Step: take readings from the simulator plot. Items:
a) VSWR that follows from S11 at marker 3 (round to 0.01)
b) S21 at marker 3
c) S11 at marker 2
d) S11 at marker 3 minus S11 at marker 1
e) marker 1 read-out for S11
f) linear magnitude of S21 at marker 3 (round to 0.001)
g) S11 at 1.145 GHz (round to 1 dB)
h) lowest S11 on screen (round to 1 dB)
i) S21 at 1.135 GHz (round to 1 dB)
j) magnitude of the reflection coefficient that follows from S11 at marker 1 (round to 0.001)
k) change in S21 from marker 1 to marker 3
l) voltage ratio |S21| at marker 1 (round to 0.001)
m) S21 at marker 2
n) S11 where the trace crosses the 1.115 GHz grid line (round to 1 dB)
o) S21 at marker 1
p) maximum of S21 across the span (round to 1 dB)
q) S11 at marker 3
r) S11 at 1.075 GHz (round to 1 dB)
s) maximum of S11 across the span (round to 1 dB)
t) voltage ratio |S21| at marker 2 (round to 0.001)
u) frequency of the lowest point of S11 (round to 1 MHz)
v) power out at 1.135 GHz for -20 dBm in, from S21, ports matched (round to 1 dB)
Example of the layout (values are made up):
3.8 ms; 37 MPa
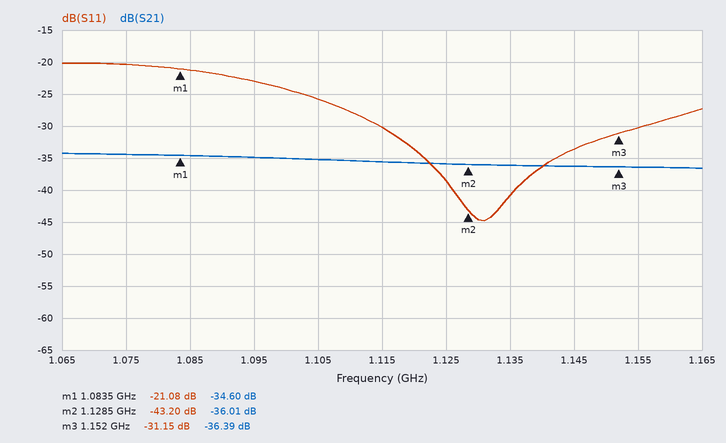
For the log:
1.06; -36.39 dB; -43.20 dB; -10.07 dB; -21.08 dB; 0.015; -34 dB; -45 dB; -36 dB; 0.088; -1.79 dB; 0.019; -36.01 dB; -30 dB; -34.60 dB; -34 dB; -31.15 dB; -20 dB; -20 dB; 0.016; 1.131 GHz; -56 dBm
